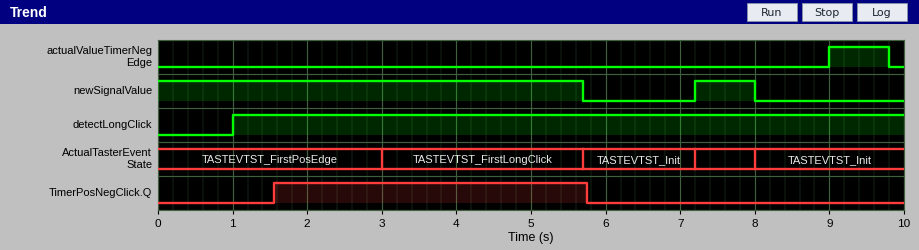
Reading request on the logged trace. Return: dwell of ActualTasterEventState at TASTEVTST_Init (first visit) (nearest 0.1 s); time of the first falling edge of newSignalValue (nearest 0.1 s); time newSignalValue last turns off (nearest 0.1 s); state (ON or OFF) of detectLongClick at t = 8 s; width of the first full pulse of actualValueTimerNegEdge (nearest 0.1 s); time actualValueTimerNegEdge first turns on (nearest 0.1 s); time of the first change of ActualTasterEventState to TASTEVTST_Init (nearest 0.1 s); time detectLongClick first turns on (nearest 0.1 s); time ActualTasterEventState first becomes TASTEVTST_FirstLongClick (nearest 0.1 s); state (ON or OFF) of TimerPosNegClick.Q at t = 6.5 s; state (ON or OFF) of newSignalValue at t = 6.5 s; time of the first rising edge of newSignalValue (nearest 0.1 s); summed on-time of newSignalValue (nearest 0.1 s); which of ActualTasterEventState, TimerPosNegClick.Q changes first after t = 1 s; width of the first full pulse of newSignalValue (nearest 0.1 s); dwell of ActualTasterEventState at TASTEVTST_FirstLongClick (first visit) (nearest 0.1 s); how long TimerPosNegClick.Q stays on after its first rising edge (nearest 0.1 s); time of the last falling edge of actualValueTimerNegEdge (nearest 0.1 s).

1.5 s
5.7 s
8.0 s
ON
0.8 s
9.0 s
5.7 s
1.0 s
3.0 s
OFF
OFF
7.2 s
6.5 s
TimerPosNegClick.Q
0.8 s
2.7 s
4.2 s
9.8 s
